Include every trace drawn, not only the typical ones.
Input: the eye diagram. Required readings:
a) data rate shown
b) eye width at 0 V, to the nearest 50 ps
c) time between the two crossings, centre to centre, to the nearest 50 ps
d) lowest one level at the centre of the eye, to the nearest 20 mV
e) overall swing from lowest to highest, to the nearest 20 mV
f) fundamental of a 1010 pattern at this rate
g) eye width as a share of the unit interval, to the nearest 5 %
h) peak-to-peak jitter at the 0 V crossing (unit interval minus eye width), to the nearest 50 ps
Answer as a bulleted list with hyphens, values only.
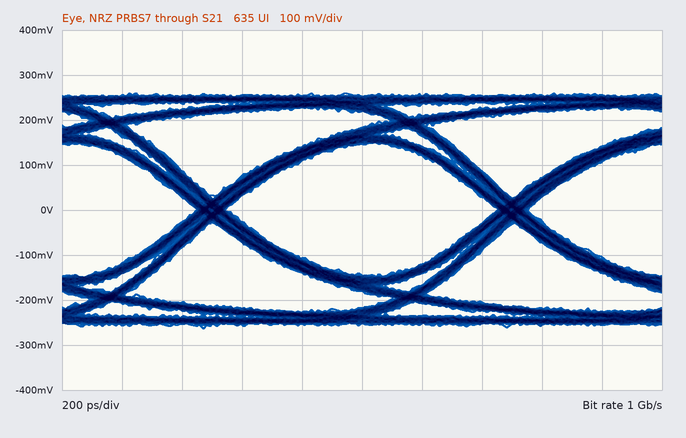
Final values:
- 1 Gb/s
- 900 ps
- 1.00 ns
- 140 mV
- 520 mV
- 500 MHz
- 90 %
- 100 ps
